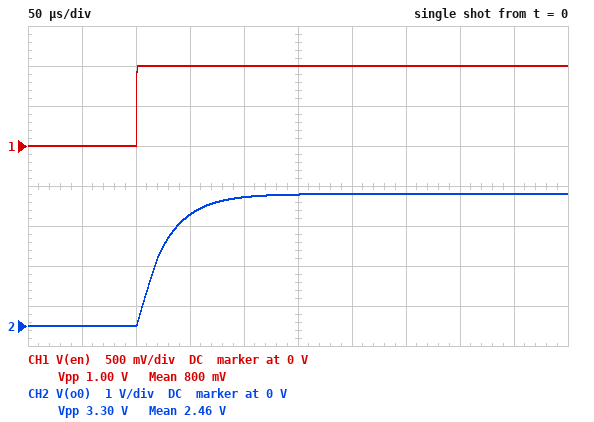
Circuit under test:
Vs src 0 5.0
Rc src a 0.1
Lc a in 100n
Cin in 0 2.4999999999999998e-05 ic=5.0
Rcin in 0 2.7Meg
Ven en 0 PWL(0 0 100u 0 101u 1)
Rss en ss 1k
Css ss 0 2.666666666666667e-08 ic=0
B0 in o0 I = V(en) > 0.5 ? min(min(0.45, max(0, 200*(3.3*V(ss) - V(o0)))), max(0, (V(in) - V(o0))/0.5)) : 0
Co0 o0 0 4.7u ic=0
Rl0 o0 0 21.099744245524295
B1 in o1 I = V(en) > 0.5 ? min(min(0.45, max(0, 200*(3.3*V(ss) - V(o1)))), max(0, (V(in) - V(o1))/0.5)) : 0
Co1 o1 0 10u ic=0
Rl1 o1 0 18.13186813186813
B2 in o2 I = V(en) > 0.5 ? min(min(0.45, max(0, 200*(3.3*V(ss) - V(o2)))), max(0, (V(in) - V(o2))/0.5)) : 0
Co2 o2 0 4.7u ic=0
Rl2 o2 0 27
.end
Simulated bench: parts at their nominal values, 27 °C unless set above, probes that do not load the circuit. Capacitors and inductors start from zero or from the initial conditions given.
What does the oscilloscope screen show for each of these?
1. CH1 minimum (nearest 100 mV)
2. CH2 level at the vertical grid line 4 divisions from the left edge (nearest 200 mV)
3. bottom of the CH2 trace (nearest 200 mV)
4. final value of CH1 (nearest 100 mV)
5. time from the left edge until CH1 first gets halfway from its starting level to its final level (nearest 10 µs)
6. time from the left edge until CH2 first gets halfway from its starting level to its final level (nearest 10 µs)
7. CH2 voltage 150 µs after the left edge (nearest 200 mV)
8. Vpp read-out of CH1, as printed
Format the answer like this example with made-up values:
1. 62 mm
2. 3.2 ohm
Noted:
1. 0 V
2. 3.2 V
3. 0 V
4. 1.0 V
5. 100 µs
6. 120 µs
7. 2.8 V
8. 1.00 V
